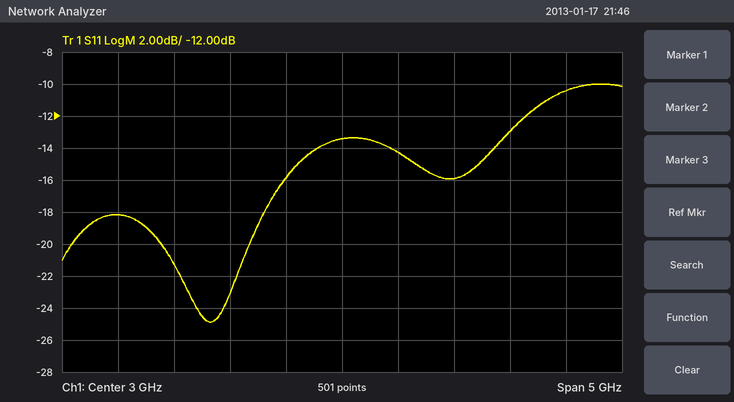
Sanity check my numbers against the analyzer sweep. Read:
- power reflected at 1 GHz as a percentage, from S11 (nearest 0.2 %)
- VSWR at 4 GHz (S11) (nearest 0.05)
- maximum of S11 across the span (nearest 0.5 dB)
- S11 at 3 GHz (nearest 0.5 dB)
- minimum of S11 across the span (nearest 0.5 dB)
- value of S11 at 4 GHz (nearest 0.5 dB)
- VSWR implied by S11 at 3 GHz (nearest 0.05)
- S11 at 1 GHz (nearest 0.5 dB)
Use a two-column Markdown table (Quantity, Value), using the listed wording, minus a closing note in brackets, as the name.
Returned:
| Quantity | Value |
|---|---|
| power reflected at 1 GHz as a percentage, from S11 | 1.6 % |
| VSWR at 4 GHz (S11) | 1.40 |
| maximum of S11 across the span | -10.0 dB |
| S11 at 3 GHz | -13.5 dB |
| minimum of S11 across the span | -25.0 dB |
| value of S11 at 4 GHz | -16.0 dB |
| VSWR implied by S11 at 3 GHz | 1.55 |
| S11 at 1 GHz | -18.0 dB |
